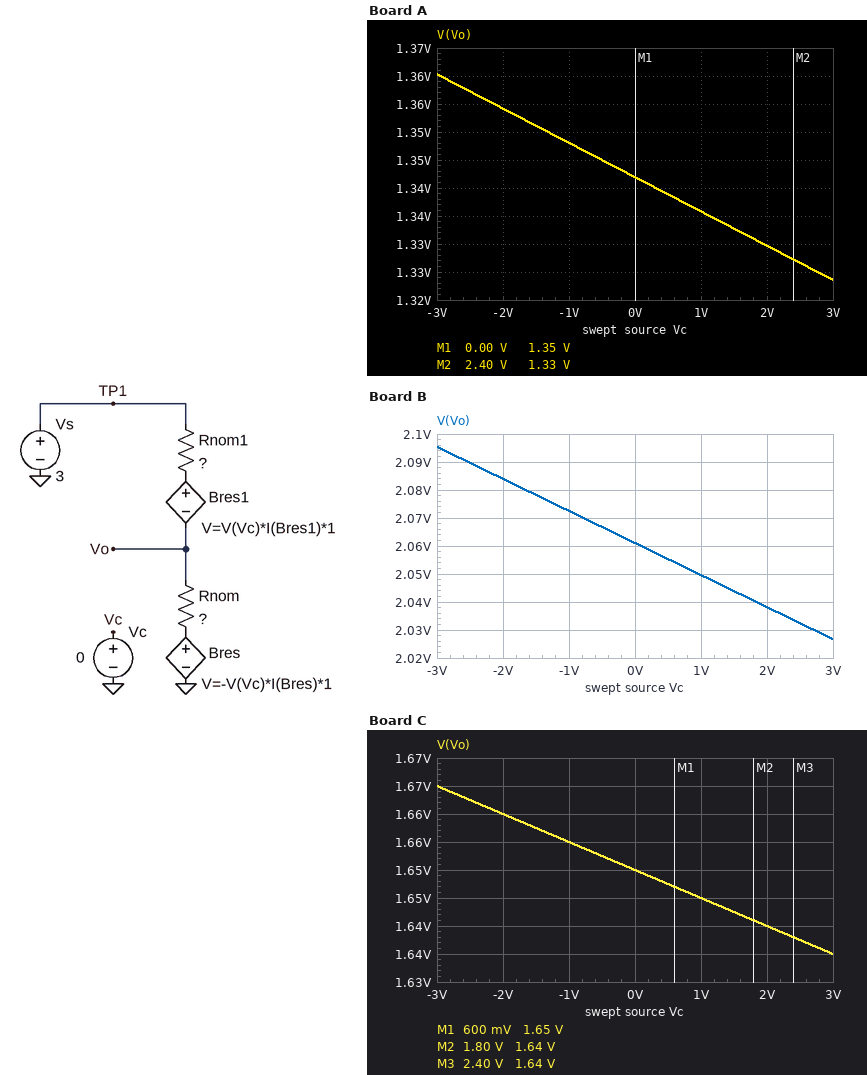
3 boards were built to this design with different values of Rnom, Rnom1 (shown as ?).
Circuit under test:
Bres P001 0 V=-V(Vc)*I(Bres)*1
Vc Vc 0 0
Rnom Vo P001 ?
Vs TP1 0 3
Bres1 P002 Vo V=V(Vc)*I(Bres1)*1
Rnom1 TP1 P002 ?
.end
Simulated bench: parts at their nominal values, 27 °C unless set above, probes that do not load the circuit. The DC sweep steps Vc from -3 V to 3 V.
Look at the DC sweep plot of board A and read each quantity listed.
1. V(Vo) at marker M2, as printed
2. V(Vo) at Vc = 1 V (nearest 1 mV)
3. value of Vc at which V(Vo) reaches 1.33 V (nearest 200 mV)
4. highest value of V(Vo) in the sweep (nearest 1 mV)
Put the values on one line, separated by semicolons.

1.33 V; 1.341 V; 2.0 V; 1.365 V
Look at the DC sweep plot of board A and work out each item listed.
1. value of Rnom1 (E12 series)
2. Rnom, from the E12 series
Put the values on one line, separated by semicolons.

270 Ω; 220 Ω
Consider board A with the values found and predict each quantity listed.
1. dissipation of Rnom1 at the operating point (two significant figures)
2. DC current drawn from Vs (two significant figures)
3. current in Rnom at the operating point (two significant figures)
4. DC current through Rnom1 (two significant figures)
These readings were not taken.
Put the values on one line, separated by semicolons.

10 mW; 6.1 mA; 6.1 mA; 6.1 mA
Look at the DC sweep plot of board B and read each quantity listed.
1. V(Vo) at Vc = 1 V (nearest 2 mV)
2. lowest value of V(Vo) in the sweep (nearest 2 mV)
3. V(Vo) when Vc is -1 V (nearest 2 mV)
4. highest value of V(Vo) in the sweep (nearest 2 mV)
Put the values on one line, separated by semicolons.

2.050 V; 2.026 V; 2.072 V; 2.096 V
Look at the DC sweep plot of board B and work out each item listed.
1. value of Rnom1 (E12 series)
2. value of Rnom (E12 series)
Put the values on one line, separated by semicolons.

82 Ω; 180 Ω
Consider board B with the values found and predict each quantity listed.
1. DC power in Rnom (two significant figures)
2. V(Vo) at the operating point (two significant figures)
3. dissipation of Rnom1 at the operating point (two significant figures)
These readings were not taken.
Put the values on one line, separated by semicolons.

24 mW; 2.1 V; 11 mW
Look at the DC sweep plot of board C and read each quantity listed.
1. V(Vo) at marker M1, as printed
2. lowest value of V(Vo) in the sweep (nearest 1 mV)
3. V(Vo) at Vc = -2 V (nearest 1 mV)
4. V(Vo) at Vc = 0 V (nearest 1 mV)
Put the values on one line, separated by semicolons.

1.65 V; 1.635 V; 1.660 V; 1.650 V
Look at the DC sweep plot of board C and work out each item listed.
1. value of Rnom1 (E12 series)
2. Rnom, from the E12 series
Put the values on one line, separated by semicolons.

270 Ω; 330 Ω
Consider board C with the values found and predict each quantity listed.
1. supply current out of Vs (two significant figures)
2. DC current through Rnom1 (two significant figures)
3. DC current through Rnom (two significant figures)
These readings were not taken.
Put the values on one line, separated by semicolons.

5.0 mA; 5.0 mA; 5.0 mA
